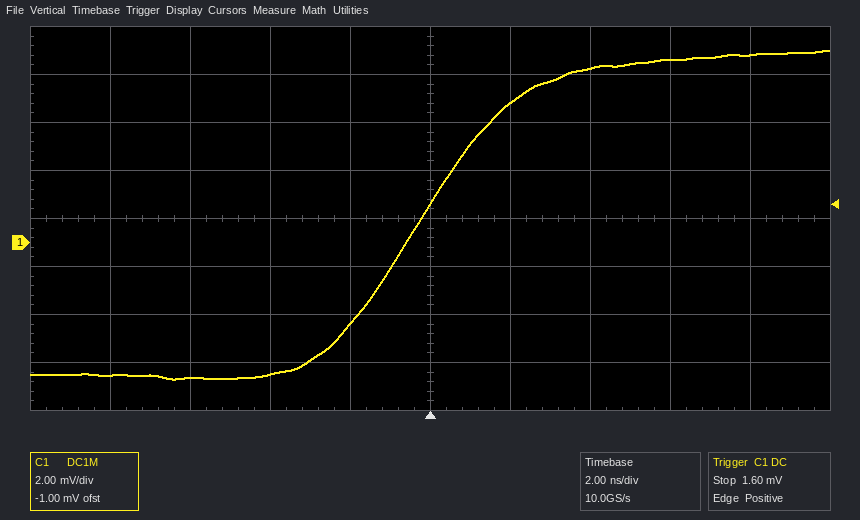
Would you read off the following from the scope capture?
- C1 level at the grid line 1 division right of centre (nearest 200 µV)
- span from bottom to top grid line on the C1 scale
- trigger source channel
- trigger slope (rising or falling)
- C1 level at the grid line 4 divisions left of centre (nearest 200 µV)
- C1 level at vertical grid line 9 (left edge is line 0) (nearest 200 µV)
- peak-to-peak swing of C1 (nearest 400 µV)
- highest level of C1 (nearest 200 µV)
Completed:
5.8 mV
16 mV
C1
rising
-5.6 mV
7.8 mV
13.6 mV
8.0 mV
